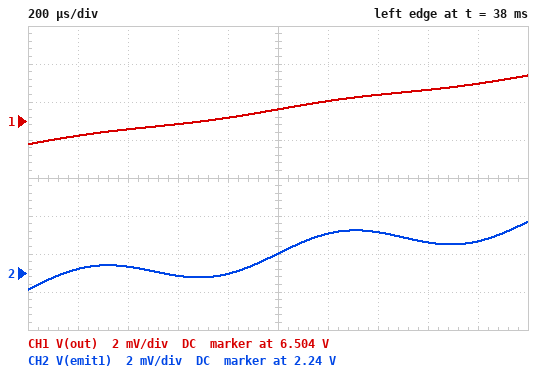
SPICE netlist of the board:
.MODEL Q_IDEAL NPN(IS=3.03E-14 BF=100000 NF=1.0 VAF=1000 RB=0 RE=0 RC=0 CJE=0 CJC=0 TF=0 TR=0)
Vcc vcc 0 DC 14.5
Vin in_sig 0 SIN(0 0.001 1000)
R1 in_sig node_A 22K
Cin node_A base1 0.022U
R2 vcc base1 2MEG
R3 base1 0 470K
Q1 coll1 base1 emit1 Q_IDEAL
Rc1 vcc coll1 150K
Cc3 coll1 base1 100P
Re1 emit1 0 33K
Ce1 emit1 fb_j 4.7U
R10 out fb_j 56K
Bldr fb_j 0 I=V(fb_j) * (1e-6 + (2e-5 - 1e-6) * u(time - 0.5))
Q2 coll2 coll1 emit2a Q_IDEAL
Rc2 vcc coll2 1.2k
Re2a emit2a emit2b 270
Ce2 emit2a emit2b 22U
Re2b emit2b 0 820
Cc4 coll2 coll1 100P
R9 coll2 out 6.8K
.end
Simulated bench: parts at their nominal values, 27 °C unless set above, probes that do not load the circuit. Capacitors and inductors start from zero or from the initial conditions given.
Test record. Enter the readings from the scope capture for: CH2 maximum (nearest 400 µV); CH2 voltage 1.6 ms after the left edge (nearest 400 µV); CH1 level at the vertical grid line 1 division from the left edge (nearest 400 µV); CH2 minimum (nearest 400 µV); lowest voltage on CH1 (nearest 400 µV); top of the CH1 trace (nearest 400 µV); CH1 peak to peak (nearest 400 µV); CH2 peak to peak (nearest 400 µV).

2.2428 V
2.2416 V
6.5032 V
2.2392 V
6.5028 V
6.5064 V
3.6 mV
3.6 mV
